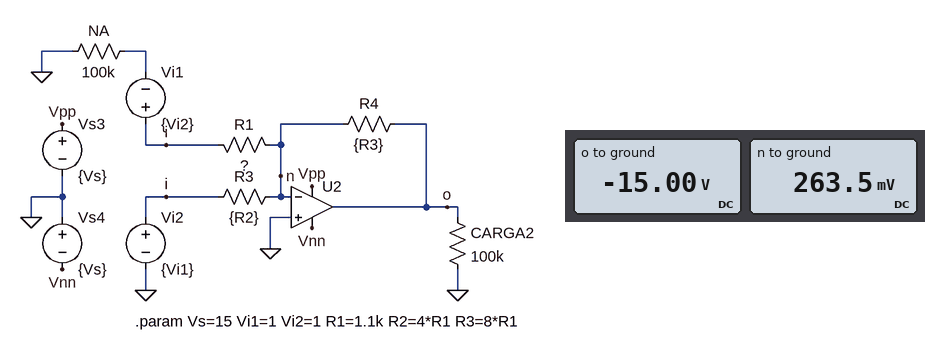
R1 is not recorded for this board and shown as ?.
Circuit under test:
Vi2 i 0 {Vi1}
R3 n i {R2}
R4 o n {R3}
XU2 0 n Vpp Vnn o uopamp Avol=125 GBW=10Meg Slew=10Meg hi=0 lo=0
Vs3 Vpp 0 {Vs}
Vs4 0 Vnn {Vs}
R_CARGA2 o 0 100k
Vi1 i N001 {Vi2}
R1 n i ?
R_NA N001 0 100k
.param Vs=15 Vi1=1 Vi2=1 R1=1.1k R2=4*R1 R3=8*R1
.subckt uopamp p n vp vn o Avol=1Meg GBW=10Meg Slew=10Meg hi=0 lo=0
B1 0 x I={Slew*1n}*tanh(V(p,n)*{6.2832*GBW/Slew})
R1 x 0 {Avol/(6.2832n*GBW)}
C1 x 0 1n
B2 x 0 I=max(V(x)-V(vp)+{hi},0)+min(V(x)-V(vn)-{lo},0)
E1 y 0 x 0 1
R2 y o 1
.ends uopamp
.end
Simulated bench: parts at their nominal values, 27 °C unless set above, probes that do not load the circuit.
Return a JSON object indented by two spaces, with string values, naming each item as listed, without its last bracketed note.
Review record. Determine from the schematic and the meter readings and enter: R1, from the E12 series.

{
  "R1, from the E12 series": "470 Ω"
}
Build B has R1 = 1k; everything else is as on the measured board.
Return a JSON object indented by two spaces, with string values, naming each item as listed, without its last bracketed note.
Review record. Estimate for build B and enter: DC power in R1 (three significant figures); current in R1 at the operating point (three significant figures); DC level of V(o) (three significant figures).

{
  "DC power in R1": "836 µW",
  "current in R1 at the operating point": "914 µA",
  "DC level of V(o)": "-9.79 V"
}
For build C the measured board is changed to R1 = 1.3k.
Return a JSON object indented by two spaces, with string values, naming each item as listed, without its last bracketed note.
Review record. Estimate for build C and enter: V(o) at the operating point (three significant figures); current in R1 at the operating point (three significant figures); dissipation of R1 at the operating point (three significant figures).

{
  "V(o) at the operating point": "-8.10 V",
  "current in R1 at the operating point": "716 µA",
  "dissipation of R1 at the operating point": "667 µW"
}
